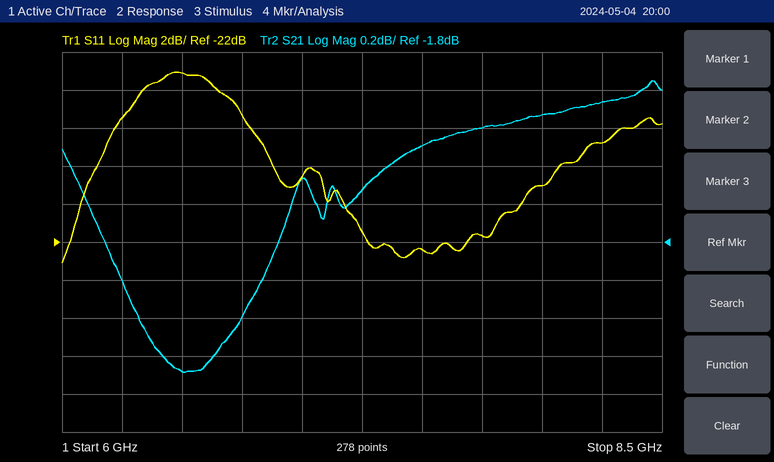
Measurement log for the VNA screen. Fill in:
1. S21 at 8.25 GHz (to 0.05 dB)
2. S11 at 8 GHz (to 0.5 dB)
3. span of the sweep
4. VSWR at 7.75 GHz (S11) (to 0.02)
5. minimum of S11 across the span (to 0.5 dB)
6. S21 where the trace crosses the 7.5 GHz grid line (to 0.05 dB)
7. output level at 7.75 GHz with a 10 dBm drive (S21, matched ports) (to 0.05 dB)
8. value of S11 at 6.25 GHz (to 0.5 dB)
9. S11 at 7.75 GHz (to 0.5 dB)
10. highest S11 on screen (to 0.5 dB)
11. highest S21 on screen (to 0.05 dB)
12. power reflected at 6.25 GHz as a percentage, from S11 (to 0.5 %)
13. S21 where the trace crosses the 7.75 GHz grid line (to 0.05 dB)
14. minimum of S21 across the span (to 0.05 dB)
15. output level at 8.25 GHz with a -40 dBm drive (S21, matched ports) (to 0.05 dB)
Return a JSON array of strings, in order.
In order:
["-1.05 dB", "-19.0 dB", "2.5 GHz", "1.18", "-23.0 dB", "-1.30 dB", "8.80 dBm", "-15.5 dB", "-21.5 dB", "-13.0 dB", "-0.95 dB", "3.0 %", "-1.20 dB", "-2.50 dB", "-41.05 dBm"]
